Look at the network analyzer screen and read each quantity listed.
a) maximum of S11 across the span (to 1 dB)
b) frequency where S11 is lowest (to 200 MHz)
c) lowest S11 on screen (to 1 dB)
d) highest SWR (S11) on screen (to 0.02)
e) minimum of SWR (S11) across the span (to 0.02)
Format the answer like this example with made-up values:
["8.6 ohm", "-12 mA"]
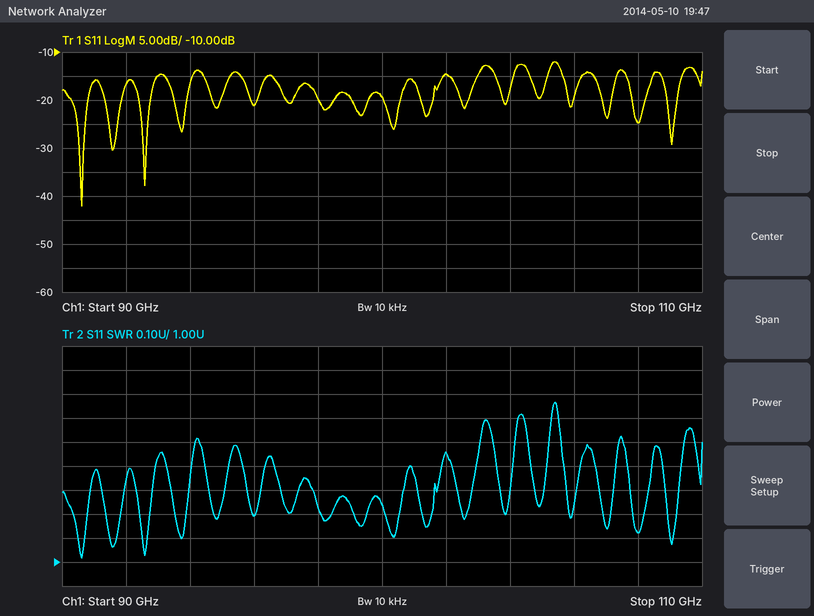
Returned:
["-12 dB", "90.6 GHz", "-42 dB", "1.66", "1.02"]
